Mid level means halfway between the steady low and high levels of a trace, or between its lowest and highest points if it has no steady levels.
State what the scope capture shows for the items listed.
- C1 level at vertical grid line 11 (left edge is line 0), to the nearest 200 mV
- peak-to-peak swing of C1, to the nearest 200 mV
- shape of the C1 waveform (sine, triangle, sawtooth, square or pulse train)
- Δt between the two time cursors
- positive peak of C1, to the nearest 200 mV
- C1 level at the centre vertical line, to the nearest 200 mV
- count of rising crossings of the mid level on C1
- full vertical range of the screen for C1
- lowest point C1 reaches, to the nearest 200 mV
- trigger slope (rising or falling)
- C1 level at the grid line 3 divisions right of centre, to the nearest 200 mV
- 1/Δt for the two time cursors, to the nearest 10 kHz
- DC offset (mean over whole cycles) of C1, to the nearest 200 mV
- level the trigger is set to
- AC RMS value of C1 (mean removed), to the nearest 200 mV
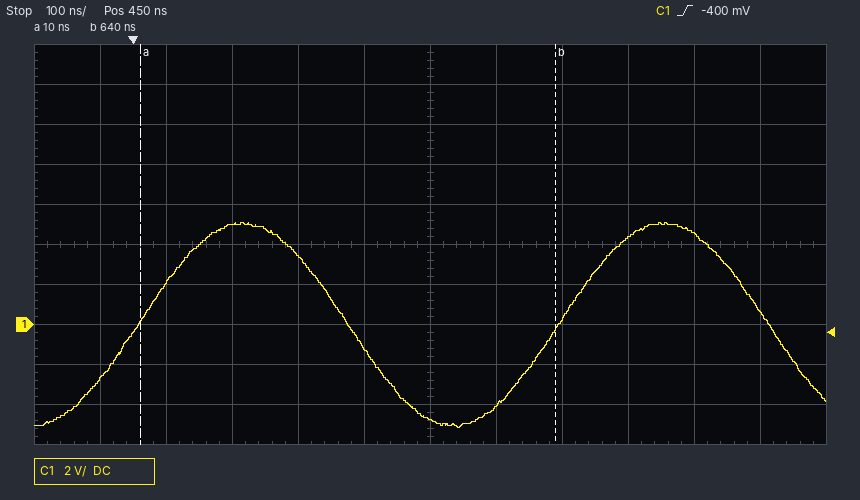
600 mV
10.2 V
sine
630 ns
5.0 V
-4.8 V
2
20 V
-5.2 V
rising
4.4 V
1.59 MHz
0.0 V
-400 mV
3.6 V
